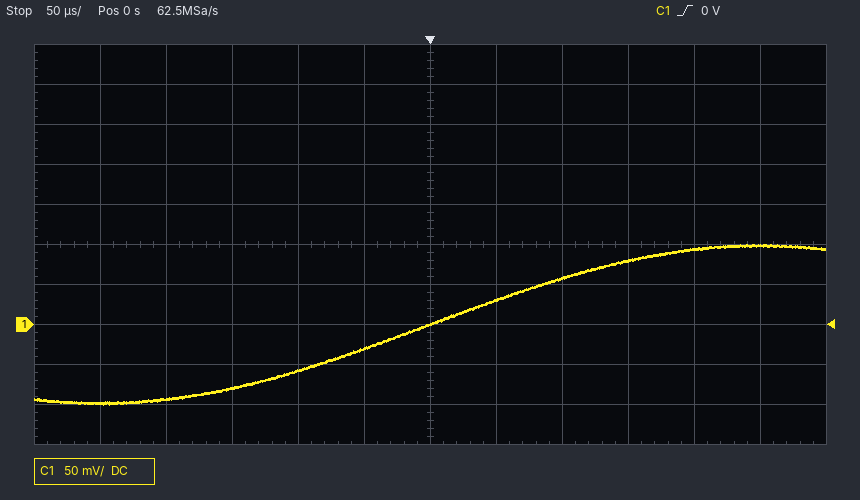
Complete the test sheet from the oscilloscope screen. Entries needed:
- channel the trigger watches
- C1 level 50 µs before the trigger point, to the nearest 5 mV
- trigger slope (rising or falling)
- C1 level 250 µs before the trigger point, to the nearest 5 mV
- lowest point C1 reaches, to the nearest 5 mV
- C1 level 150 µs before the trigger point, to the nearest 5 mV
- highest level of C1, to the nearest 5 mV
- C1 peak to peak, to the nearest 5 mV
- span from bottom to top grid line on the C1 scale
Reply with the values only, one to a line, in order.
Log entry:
C1
-30 mV
rising
-100 mV
-100 mV
-80 mV
100 mV
200 mV
500 mV
